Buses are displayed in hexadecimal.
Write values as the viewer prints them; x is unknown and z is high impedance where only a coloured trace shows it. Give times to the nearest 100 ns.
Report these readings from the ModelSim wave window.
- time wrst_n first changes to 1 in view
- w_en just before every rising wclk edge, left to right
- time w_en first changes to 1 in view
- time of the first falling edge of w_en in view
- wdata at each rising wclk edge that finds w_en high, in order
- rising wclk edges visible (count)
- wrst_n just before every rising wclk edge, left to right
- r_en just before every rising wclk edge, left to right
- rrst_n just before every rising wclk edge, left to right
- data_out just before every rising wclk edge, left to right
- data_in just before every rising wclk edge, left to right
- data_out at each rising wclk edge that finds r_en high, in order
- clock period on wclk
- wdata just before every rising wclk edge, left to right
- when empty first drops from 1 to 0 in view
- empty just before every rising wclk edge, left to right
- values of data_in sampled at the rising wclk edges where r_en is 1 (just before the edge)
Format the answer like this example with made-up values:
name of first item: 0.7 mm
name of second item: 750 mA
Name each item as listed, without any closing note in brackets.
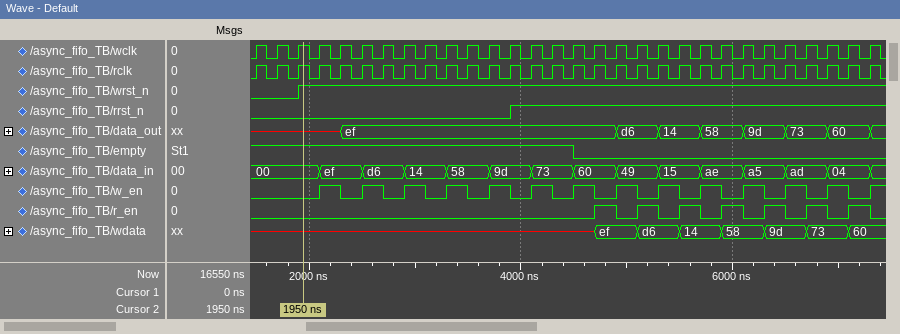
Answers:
time wrst_n first changes to 1 in view: 1900 ns
w_en just before every rising wclk edge, left to right: 0 0 0 0 1 0 1 0 1 0 1 0 1 0 1 0 1 0 1 0 1 0 1 0 1 0 1 0 1 0
time w_en first changes to 1 in view: 2100 ns
time of the first falling edge of w_en in view: 2300 ns
wdata at each rising wclk edge that finds w_en high, in order: x, x, x, x, x, x, x, ef, d6, 14, 58, 9d, 73
rising wclk edges visible: 30
wrst_n just before every rising wclk edge, left to right: 0 0 0 1 1 1 1 1 1 1 1 1 1 1 1 1 1 1 1 1 1 1 1 1 1 1 1 1 1 1
r_en just before every rising wclk edge, left to right: 0 0 0 0 0 0 0 0 0 0 0 0 0 0 0 0 0 1 0 1 0 1 0 1 0 1 0 1 0 1
rrst_n just before every rising wclk edge, left to right: 0 0 0 0 0 0 0 0 0 0 0 0 0 1 1 1 1 1 1 1 1 1 1 1 1 1 1 1 1 1
data_out just before every rising wclk edge, left to right: x, x, x, x, x, ef, ef, ef, ef, ef, ef, ef, ef, ef, ef, ef, ef, ef, d6, d6, 14, 14, 58, 58, 9d, 9d, 73, 73, 60, 60
data_in just before every rising wclk edge, left to right: 00, 00, 00, 00, ef, ef, d6, d6, 14, 14, 58, 58, 9d, 9d, 73, 73, 60, 60, 49, 49, 15, 15, ae, ae, a5, a5, ad, ad, 04, 04
data_out at each rising wclk edge that finds r_en high, in order: ef, d6, 14, 58, 9d, 73, 60
clock period on wclk: 200 ns
wdata just before every rising wclk edge, left to right: x, x, x, x, x, x, x, x, x, x, x, x, x, x, x, x, x, ef, ef, d6, d6, 14, 14, 58, 58, 9d, 9d, 73, 73, 60
when empty first drops from 1 to 0 in view: 4500 ns
empty just before every rising wclk edge, left to right: 1 1 1 1 1 1 1 1 1 1 1 1 1 1 1 1 0 0 0 0 0 0 0 0 0 0 0 0 0 0
values of data_in sampled at the rising wclk edges where r_en is 1: 60, 49, 15, ae, a5, ad, 04
